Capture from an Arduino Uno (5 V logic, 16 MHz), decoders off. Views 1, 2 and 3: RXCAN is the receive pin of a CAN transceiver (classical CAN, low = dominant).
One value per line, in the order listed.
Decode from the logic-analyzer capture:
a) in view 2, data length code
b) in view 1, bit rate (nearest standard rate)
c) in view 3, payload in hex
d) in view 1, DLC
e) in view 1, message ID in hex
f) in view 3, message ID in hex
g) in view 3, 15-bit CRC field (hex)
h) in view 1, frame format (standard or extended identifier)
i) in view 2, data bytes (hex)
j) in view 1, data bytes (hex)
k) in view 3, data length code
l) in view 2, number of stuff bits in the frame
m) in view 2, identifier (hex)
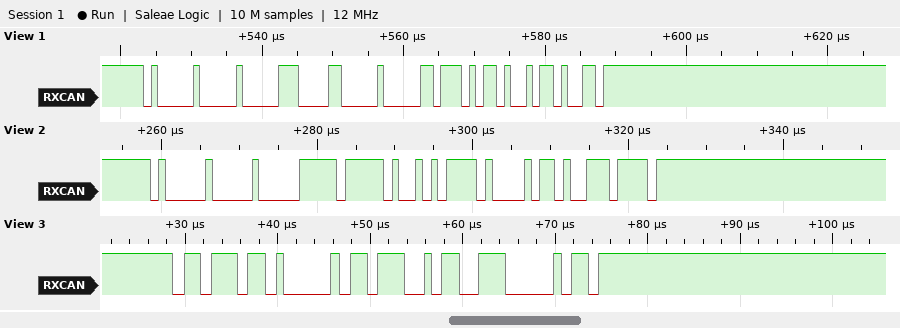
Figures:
3
1000 kbit/s
B9
3
0x400
0x6ED
0x3381
standard
FF 2B D0
0C 00 BA
1
5
0x400
